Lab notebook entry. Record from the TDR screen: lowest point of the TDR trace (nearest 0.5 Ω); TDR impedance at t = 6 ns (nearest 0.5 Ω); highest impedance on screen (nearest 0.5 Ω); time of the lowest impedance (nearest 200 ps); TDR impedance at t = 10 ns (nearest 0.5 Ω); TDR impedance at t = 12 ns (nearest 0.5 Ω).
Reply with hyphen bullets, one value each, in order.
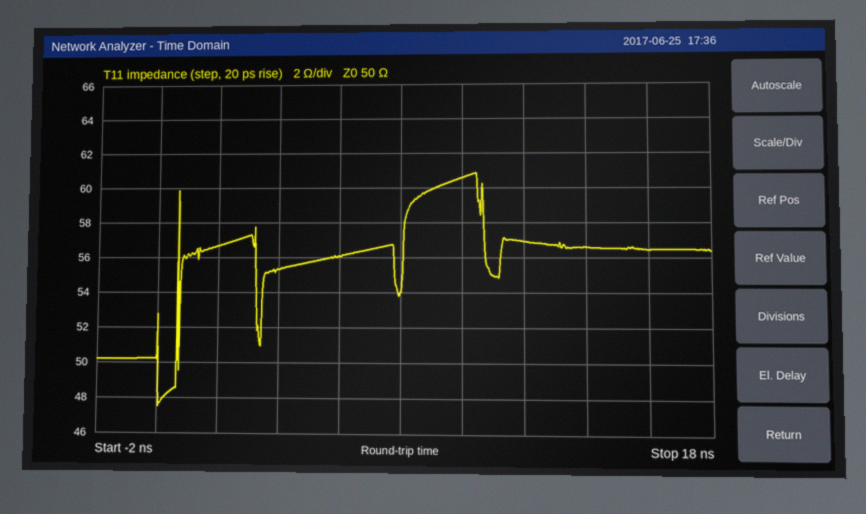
- 47.5 Ω
- 56.0 Ω
- 61.0 Ω
- 0.0 ns
- 60.5 Ω
- 57.0 Ω
